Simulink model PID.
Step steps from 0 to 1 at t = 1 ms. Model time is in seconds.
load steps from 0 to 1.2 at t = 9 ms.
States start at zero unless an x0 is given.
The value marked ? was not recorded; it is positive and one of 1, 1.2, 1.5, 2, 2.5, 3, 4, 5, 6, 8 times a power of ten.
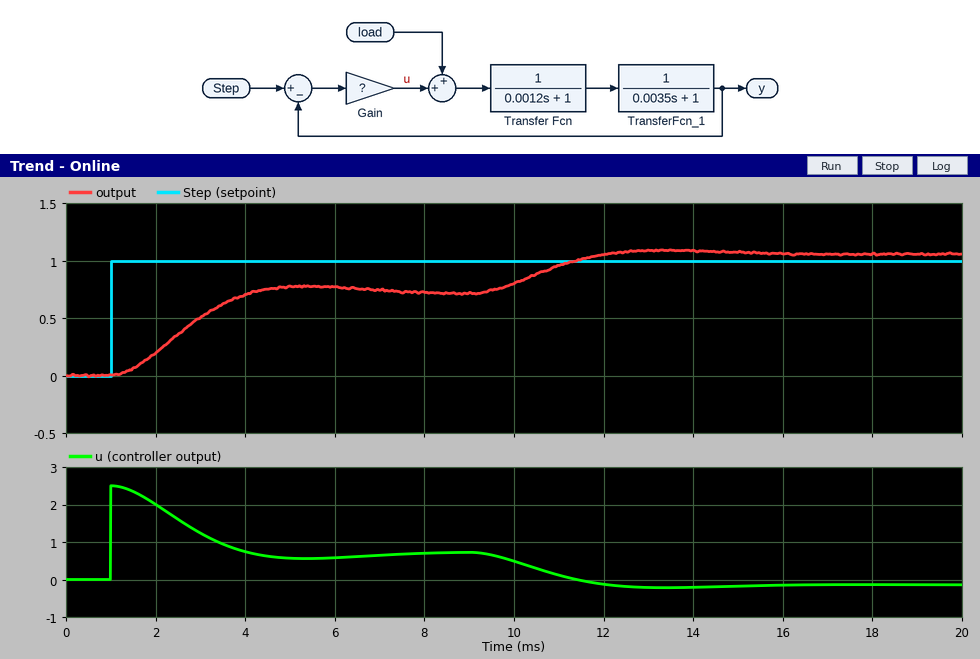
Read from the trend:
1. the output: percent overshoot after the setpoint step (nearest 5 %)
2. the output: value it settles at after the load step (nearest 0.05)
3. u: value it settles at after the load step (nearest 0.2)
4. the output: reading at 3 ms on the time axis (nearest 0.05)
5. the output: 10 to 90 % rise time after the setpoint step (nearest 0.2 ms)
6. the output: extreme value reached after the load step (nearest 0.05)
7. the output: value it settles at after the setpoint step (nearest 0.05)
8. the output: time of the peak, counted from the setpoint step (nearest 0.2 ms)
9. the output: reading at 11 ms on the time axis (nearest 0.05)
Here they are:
10 %
1.05
-0.2
0.50
2.0 ms
1.10
0.70
4.4 ms
0.95
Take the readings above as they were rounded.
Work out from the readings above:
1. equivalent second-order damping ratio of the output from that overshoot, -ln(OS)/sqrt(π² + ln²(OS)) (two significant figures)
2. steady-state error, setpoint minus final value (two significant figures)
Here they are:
0.59
0.30
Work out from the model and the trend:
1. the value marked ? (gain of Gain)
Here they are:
2.5
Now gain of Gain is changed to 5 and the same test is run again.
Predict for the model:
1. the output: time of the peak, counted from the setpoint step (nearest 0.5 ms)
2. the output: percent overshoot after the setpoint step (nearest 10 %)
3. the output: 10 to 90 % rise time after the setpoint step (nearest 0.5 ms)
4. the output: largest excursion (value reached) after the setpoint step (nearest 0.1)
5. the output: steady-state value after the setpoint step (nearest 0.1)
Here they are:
3.0 ms
20 %
1.5 ms
1.0
0.8
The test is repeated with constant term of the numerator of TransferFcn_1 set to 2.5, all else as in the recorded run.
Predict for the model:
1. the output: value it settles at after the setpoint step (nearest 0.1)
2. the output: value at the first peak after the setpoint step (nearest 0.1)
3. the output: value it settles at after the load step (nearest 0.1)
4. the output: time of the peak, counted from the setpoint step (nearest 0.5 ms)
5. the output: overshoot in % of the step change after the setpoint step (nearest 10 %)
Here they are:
0.9
1.1
1.3
2.5 ms
20 %
